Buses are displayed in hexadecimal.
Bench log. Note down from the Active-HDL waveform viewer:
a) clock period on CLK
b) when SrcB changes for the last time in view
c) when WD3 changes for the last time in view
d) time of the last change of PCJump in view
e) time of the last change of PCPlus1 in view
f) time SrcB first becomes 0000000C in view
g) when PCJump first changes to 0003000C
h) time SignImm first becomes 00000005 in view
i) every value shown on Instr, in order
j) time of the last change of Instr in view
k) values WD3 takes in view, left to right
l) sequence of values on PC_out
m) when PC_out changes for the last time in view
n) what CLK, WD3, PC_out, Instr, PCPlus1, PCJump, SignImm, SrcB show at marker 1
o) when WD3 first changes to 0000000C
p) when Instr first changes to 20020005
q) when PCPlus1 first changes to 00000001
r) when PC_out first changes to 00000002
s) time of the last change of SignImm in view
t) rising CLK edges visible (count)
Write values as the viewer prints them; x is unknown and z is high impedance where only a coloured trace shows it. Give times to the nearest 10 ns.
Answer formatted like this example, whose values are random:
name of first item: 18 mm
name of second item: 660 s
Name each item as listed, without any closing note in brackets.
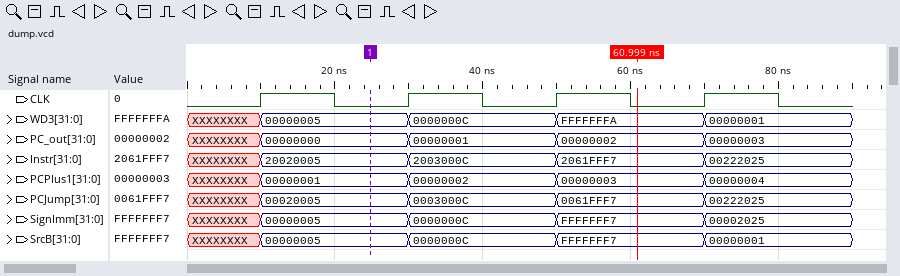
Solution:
clock period on CLK: 20 ns
when SrcB changes for the last time in view: 70 ns
when WD3 changes for the last time in view: 70 ns
time of the last change of PCJump in view: 70 ns
time of the last change of PCPlus1 in view: 70 ns
time SrcB first becomes 0000000C in view: 30 ns
when PCJump first changes to 0003000C: 30 ns
time SignImm first becomes 00000005 in view: 10 ns
every value shown on Instr, in order: XXXXXXXX, 20020005, 2003000C, 2061FFF7, 00222025
time of the last change of Instr in view: 70 ns
values WD3 takes in view, left to right: XXXXXXXX, 00000005, 0000000C, FFFFFFFA, 00000001
sequence of values on PC_out: XXXXXXXX, 00000000, 00000001, 00000002, 00000003
when PC_out changes for the last time in view: 70 ns
what CLK, WD3, PC_out, Instr, PCPlus1, PCJump, SignImm, SrcB show at marker 1: CLK=0, WD3=00000005, PC_out=00000000, Instr=20020005, PCPlus1=00000001, PCJump=00020005, SignImm=00000005, SrcB=00000005
when WD3 first changes to 0000000C: 30 ns
when Instr first changes to 20020005: 10 ns
when PCPlus1 first changes to 00000001: 10 ns
when PC_out first changes to 00000002: 50 ns
time of the last change of SignImm in view: 70 ns
rising CLK edges visible: 4
